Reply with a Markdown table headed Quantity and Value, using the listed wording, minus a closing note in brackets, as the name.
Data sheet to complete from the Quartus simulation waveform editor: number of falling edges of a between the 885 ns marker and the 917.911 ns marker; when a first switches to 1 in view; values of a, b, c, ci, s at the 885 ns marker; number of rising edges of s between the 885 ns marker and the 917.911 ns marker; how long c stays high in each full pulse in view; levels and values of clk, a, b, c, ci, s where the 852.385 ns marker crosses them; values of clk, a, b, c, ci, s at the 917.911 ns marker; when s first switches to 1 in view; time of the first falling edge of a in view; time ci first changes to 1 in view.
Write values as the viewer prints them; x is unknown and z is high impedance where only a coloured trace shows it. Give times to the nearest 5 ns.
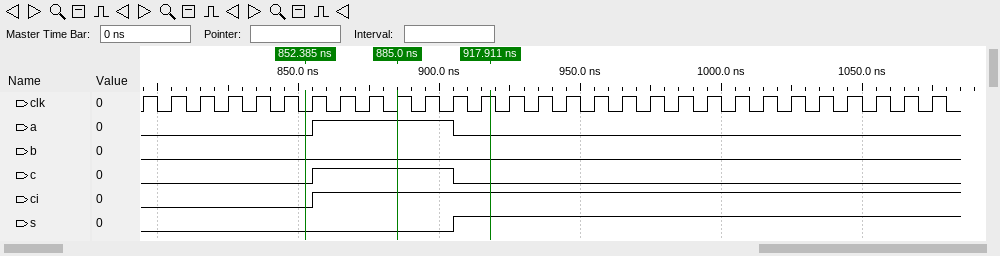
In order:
| Quantity | Value |
|---|---|
| number of falling edges of a between the 885 ns marker and the 917.911 ns marker | 1 |
| when a first switches to 1 in view | 855 ns |
| values of a, b, c, ci, s at the 885 ns marker | a=1, b=0, c=1, ci=1, s=0 |
| number of rising edges of s between the 885 ns marker and the 917.911 ns marker | 1 |
| how long c stays high in each full pulse in view | 50 ns |
| levels and values of clk, a, b, c, ci, s where the 852.385 ns marker crosses them | clk=0, a=0, b=0, c=0, ci=0, s=0 |
| values of clk, a, b, c, ci, s at the 917.911 ns marker | clk=1, a=0, b=0, c=0, ci=1, s=1 |
| when s first switches to 1 in view | 905 ns |
| time of the first falling edge of a in view | 905 ns |
| time ci first changes to 1 in view | 855 ns |
